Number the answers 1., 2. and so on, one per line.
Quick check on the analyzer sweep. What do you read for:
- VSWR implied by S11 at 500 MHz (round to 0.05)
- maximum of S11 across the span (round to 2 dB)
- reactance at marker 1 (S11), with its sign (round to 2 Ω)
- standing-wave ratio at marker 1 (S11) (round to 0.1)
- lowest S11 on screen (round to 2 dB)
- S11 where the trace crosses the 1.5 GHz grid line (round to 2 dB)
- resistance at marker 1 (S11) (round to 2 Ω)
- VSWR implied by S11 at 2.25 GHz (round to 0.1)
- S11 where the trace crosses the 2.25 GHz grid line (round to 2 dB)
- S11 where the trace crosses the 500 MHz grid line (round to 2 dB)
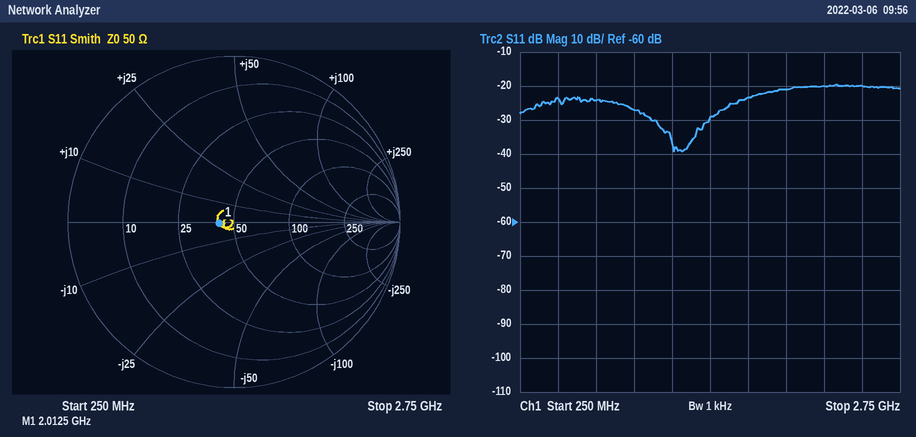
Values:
1. 1.15
2. -20 dB
3. 0 Ω
4. 1.2
5. -40 dB
6. -30 dB
7. 42 Ω
8. 1.2
9. -20 dB
10. -24 dB
